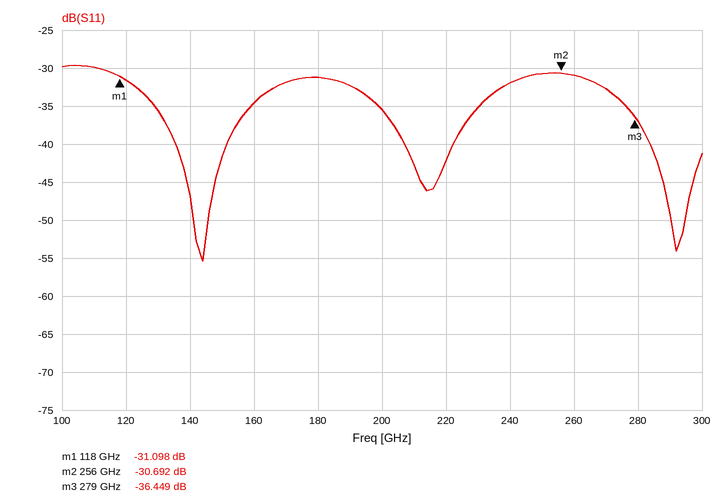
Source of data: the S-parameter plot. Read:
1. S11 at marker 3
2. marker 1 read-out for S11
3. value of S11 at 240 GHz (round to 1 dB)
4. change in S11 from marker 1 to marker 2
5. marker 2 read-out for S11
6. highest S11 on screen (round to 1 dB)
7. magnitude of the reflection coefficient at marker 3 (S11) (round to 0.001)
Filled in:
-36.449 dB
-31.098 dB
-32 dB
0.406 dB
-30.692 dB
-30 dB
0.015
